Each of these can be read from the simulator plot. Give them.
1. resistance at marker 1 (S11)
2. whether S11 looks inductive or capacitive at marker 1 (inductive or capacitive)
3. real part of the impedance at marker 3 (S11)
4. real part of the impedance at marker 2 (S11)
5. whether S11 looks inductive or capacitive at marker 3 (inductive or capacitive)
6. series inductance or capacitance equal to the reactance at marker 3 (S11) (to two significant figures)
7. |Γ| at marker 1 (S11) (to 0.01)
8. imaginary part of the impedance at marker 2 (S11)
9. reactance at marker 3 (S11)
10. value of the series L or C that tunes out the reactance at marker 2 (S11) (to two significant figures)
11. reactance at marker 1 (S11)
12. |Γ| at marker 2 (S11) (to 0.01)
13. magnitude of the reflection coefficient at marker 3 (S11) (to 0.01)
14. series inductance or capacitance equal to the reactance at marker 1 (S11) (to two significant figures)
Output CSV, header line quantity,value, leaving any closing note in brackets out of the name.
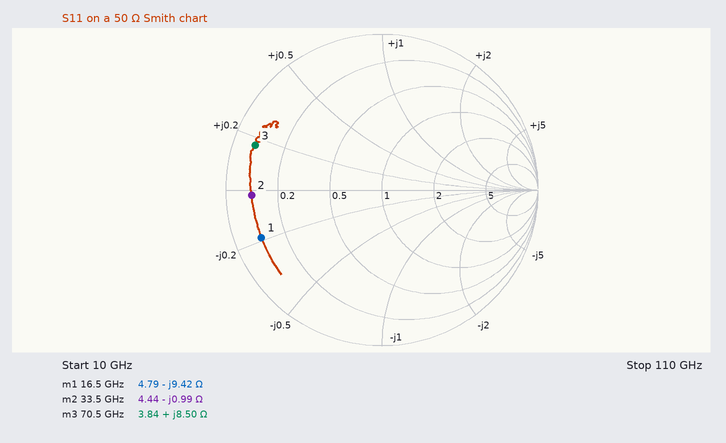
quantity,value
resistance at marker 1,4.79 Ω
whether S11 looks inductive or capacitive at marker 1,capacitive
real part of the impedance at marker 3,3.84 Ω
real part of the impedance at marker 2,4.44 Ω
whether S11 looks inductive or capacitive at marker 3,inductive
series inductance or capacitance equal to the reactance at marker 3 (S11),19 pH
|Γ| at marker 1 (S11),0.83
imaginary part of the impedance at marker 2,-0.99 Ω
reactance at marker 3,+8.50 Ω
value of the series L or C that tunes out the reactance at marker 2 (S11),4.7 pH
reactance at marker 1,-9.42 Ω
|Γ| at marker 2 (S11),0.84
magnitude of the reflection coefficient at marker 3 (S11),0.86
series inductance or capacitance equal to the reactance at marker 1 (S11),1.0 pF
